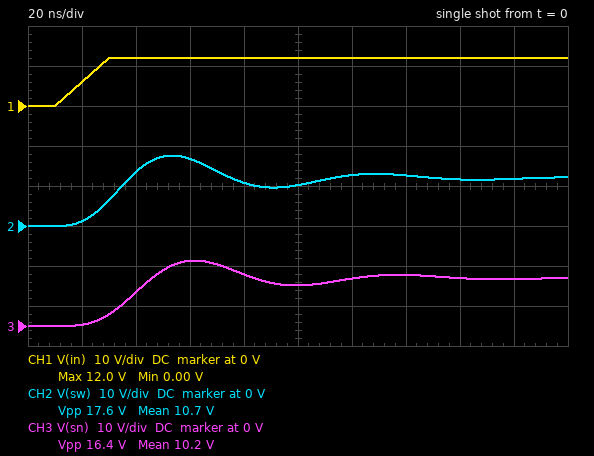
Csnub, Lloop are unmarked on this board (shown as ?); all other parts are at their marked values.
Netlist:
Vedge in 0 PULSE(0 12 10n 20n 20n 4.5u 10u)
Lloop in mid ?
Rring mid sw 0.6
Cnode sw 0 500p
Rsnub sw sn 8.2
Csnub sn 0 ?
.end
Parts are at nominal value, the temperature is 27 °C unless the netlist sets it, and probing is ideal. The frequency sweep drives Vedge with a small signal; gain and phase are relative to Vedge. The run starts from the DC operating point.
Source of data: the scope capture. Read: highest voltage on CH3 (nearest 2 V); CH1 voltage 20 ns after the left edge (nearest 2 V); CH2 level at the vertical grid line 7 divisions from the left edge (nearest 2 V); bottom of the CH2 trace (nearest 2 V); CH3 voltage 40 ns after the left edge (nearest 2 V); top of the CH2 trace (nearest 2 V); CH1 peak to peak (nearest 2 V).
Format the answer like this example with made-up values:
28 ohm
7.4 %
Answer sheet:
16 V
6 V
12 V
0 V
8 V
18 V
12 V
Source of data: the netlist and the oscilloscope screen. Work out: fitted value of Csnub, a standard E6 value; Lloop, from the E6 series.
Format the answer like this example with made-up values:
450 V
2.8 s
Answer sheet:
1 nF
100 nH
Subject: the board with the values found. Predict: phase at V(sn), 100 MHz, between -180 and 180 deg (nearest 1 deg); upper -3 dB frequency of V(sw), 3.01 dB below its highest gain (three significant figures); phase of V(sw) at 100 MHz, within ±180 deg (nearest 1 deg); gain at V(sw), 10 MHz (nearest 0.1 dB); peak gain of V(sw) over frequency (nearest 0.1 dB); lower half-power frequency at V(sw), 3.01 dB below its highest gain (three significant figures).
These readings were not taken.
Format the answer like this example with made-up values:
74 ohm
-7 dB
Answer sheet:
122 deg
16.5 MHz
-159 deg
5.2 dB
7.3 dB
9.03 MHz
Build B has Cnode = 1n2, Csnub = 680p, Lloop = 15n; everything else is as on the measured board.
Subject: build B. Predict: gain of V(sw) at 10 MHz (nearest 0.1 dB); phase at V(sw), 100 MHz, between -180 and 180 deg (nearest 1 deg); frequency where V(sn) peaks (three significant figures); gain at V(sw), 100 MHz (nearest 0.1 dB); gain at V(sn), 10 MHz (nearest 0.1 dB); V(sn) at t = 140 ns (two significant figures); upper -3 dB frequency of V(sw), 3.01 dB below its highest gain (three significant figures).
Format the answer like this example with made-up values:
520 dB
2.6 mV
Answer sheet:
0.9 dB
-166 deg
30.8 MHz
-16.3 dB
0.4 dB
12 V
39.4 MHz
